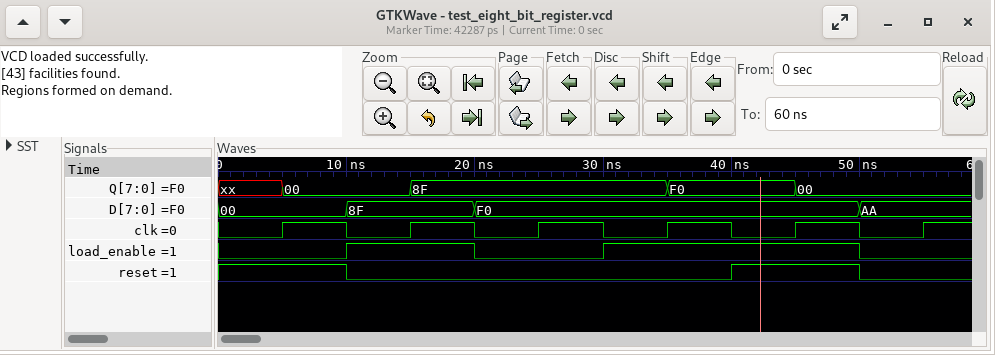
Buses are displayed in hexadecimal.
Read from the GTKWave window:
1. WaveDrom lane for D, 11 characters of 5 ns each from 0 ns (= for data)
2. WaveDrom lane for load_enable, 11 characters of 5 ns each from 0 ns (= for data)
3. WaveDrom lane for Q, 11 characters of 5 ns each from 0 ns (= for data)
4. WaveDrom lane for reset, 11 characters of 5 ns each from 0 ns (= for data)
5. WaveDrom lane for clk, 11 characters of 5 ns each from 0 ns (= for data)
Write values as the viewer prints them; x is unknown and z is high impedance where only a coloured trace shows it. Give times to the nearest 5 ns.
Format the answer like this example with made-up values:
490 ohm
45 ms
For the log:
{name: 'D', wave: '=.=.=.....=', data: '00 8F F0 AA'}
{name: 'load_enable', wave: '0.1.0.1...0'}
{name: 'Q', wave: 'x=.=...=.=.', data: '00 8F F0 00'}
{name: 'reset', wave: '1.0.....1.0'}
{name: 'clk', wave: '01010101010'}
